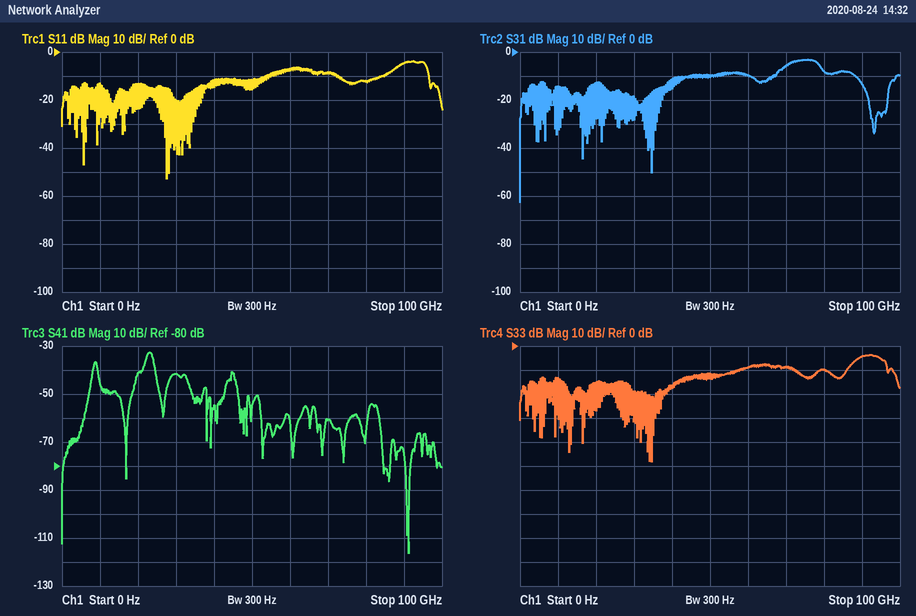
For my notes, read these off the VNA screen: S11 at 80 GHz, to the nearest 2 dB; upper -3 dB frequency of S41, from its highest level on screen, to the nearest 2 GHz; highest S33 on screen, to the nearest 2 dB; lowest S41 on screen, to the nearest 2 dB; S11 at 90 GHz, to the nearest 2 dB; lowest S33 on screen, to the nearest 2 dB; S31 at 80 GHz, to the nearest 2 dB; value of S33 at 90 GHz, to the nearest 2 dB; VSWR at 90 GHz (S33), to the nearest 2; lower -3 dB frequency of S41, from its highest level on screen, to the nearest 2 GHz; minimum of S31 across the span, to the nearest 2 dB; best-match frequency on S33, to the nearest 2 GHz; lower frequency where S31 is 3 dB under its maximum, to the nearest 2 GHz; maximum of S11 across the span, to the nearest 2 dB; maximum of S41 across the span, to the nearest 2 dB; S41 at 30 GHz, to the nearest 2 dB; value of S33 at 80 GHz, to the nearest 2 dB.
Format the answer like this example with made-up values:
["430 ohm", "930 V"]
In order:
["-12 dB", "24 GHz", "-4 dB", "-116 dB", "-4 dB", "-48 dB", "-8 dB", "-4 dB", "4", "22 GHz", "-62 dB", "34 GHz", "70 GHz", "-4 dB", "-32 dB", "-42 dB", "-10 dB"]
